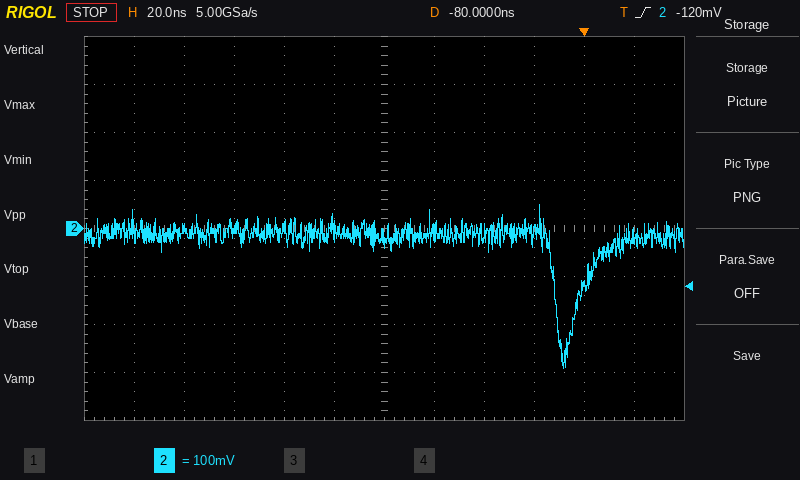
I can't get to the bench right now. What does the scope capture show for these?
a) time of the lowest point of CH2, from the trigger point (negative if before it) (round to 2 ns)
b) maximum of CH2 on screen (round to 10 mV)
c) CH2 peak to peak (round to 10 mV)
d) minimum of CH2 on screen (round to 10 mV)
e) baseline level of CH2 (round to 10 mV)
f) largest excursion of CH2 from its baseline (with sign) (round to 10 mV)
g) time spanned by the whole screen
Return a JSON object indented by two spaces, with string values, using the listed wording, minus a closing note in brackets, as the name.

{
  "time of the lowest point of CH2, from the trigger point (negative if before it)": "-8 ns",
  "maximum of CH2 on screen": "50 mV",
  "CH2 peak to peak": "340 mV",
  "minimum of CH2 on screen": "-290 mV",
  "baseline level of CH2": "-10 mV",
  "largest excursion of CH2 from its baseline (with sign)": "-280 mV",
  "time spanned by the whole screen": "240 ns"
}
